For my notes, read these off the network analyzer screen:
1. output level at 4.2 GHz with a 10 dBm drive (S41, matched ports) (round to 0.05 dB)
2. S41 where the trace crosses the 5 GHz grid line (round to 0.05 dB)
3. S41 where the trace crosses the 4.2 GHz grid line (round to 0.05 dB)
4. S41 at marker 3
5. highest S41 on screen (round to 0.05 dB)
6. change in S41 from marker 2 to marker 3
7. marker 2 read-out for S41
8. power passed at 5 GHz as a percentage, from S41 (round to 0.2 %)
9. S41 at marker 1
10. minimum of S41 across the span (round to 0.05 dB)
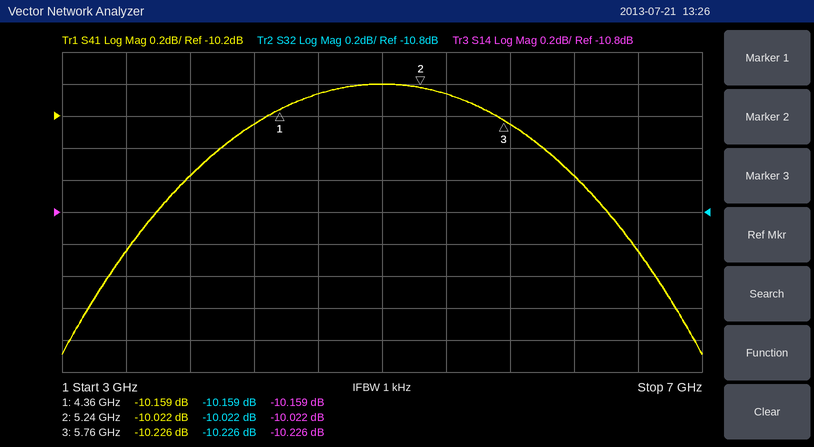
-0.25 dBm
-10.00 dB
-10.25 dB
-10.226 dB
-10.00 dB
-0.204 dB
-10.022 dB
10.0 %
-10.159 dB
-11.70 dB
